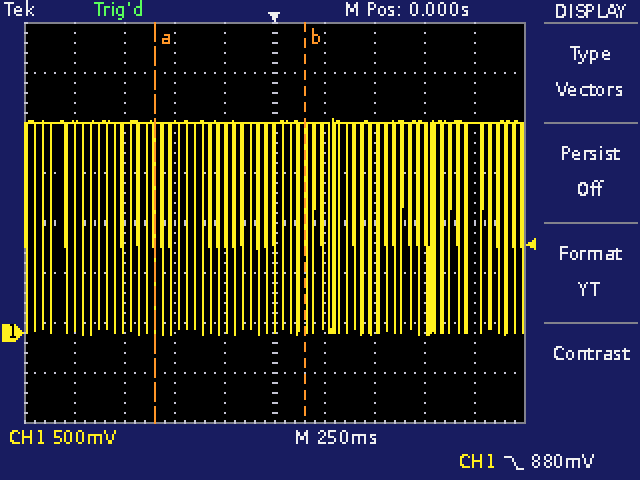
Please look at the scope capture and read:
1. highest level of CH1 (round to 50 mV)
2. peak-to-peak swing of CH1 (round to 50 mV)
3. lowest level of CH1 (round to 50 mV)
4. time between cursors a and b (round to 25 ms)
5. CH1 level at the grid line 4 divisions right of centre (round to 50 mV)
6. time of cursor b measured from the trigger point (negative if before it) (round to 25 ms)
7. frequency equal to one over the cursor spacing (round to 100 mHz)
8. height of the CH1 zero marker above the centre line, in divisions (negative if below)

2.15 V
2.15 V
0 mV
750 ms
2.10 V
+150 ms
1.3 Hz
-2.2 div
